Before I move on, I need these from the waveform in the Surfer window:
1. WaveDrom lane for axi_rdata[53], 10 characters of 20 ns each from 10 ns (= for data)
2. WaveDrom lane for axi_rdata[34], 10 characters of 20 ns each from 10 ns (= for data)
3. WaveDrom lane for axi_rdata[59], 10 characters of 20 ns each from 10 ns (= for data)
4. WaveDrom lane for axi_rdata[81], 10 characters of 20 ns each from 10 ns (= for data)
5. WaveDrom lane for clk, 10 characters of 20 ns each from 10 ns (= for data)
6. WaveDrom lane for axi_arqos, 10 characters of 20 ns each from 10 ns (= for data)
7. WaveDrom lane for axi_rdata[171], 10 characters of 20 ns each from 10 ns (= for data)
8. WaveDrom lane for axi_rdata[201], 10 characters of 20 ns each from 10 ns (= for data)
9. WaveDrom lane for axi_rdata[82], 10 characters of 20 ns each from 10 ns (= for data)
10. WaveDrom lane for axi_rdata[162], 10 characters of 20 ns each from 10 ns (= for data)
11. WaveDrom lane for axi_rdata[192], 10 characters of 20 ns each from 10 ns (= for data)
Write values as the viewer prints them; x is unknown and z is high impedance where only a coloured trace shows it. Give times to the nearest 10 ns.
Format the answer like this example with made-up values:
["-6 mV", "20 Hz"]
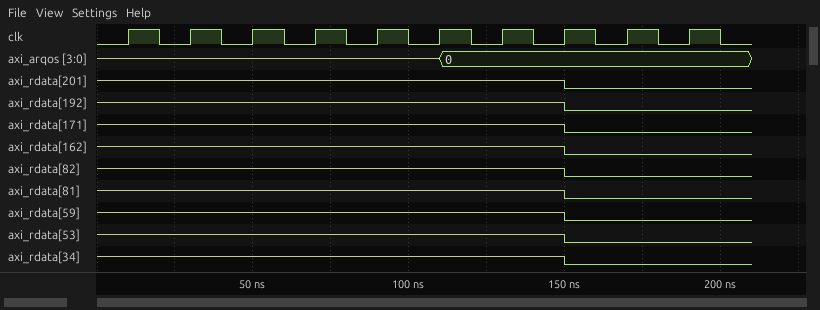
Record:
["{name: 'axi_rdata[53]', wave: 'z......0..'}", "{name: 'axi_rdata[34]', wave: 'z......0..'}", "{name: 'axi_rdata[59]', wave: 'z......0..'}", "{name: 'axi_rdata[81]', wave: 'z......0..'}", "{name: 'clk', wave: 'p.........'}", "{name: 'axi_arqos', wave: 'z....=....', data: '0'}", "{name: 'axi_rdata[171]', wave: 'z......0..'}", "{name: 'axi_rdata[201]', wave: 'z......0..'}", "{name: 'axi_rdata[82]', wave: 'z......0..'}", "{name: 'axi_rdata[162]', wave: 'z......0..'}", "{name: 'axi_rdata[192]', wave: 'z......0..'}"]
